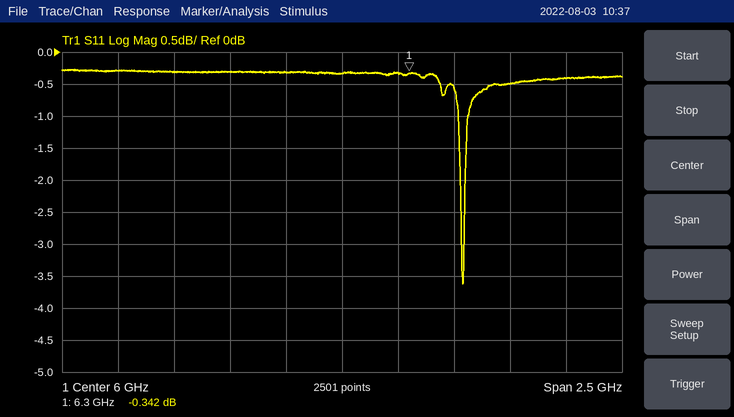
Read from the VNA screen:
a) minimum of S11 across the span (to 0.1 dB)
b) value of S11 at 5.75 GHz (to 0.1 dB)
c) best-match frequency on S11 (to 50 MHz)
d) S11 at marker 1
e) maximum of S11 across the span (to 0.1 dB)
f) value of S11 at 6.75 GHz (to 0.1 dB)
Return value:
-3.6 dB
-0.3 dB
6.55 GHz
-0.342 dB
-0.3 dB
-0.5 dB
